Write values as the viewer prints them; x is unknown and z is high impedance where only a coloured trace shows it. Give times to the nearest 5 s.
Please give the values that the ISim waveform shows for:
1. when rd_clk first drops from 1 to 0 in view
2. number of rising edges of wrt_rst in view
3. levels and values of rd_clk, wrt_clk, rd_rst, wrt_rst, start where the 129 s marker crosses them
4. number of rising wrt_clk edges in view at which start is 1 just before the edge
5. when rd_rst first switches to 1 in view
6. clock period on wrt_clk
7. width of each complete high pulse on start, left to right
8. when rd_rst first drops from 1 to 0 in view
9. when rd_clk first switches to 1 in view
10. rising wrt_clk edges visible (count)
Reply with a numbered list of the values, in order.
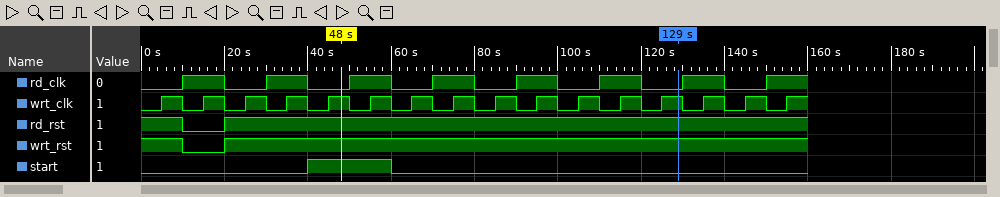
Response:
1. 20 s
2. 1
3. rd_clk=0, wrt_clk=1, rd_rst=1, wrt_rst=1, start=0
4. 2
5. 20 s
6. 10 s
7. 20 s
8. 10 s
9. 10 s
10. 16
